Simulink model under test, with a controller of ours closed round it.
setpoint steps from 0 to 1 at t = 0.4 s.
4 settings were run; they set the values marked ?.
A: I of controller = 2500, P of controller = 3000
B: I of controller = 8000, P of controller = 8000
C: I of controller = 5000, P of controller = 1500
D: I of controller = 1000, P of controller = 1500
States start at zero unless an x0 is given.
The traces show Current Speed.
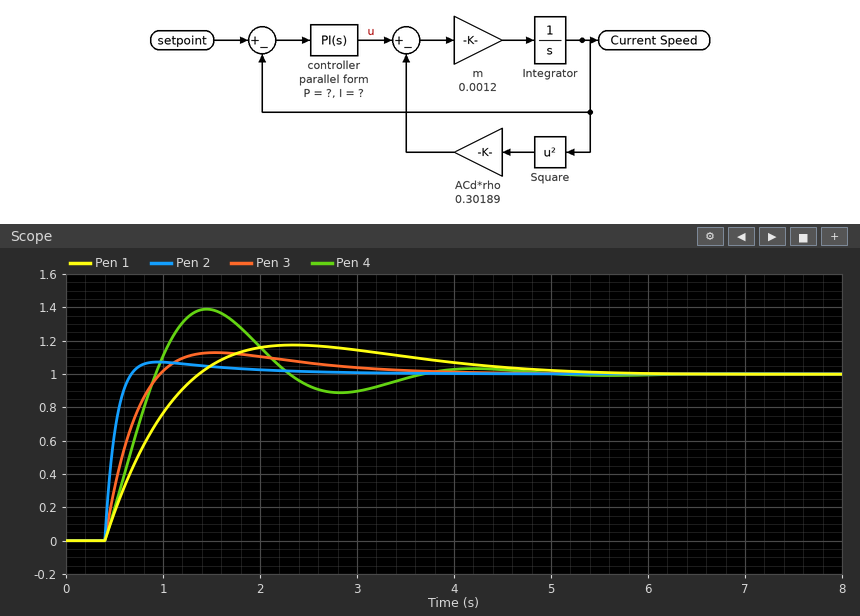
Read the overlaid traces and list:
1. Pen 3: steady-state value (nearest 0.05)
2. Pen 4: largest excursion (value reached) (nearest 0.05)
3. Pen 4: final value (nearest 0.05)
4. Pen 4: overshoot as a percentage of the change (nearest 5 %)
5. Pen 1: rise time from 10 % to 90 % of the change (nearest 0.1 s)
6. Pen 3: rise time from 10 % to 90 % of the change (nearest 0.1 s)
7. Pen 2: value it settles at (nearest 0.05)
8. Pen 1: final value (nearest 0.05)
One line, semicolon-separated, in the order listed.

1.00; 1.40; 1.00; 40 %; 0.7 s; 0.4 s; 1.00; 1.00
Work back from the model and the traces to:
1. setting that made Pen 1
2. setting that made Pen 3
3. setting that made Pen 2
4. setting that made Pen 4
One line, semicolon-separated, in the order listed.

D; A; B; C
